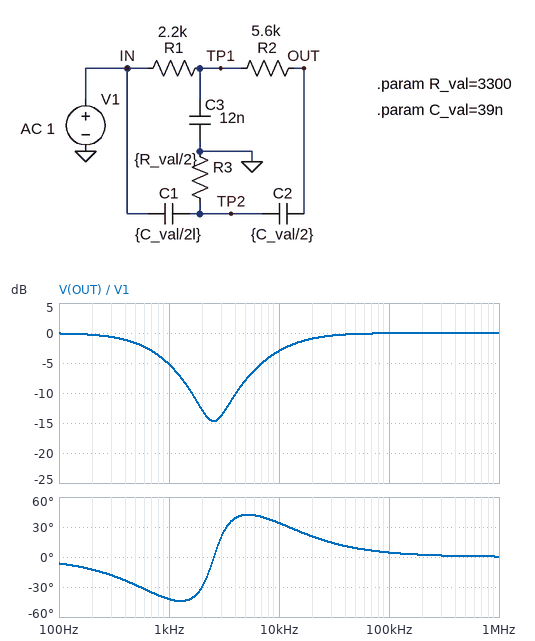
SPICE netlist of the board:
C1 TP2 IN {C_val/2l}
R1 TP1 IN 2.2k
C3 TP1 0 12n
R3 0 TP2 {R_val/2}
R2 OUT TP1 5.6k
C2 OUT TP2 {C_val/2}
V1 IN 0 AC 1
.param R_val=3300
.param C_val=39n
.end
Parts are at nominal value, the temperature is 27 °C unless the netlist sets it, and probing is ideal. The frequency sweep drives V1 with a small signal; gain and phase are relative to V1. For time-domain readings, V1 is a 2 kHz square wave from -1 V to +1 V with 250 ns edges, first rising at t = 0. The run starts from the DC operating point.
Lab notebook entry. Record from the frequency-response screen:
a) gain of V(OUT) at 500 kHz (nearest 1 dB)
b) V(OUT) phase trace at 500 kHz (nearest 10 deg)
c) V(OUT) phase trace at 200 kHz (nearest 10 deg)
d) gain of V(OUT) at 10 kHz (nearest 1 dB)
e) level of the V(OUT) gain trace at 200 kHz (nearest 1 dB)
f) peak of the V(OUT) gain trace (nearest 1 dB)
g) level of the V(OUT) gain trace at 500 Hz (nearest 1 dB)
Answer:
0 dB
0 deg
0 deg
-3 dB
0 dB
0 dB
-2 dB
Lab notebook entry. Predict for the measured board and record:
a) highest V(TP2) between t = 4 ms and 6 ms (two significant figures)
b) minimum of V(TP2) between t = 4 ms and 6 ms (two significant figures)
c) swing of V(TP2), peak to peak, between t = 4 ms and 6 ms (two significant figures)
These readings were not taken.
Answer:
1.9 V
-1.9 V
3.8 V
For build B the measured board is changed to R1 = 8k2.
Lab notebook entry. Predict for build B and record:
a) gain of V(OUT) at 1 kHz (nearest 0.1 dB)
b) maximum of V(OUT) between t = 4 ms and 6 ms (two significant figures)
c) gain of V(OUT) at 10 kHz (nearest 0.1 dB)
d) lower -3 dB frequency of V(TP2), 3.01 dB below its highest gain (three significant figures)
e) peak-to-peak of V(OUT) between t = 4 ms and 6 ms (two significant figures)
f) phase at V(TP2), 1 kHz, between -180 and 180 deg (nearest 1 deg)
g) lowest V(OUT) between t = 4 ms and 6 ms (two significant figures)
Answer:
-11.1 dB
1.7 V
-2.4 dB
7.09 kHz
3.4 V
55 deg
-1.7 V
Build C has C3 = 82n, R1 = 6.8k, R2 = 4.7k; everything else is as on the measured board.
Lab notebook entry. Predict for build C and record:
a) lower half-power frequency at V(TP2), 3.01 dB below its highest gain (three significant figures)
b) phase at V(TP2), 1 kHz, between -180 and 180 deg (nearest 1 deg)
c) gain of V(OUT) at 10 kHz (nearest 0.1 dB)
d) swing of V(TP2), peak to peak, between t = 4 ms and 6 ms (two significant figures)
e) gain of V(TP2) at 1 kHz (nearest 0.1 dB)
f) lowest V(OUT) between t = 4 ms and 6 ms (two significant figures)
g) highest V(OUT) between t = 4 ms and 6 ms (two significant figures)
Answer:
7.18 kHz
61 deg
-2.1 dB
3.9 V
-15.0 dB
-1.9 V
1.9 V
